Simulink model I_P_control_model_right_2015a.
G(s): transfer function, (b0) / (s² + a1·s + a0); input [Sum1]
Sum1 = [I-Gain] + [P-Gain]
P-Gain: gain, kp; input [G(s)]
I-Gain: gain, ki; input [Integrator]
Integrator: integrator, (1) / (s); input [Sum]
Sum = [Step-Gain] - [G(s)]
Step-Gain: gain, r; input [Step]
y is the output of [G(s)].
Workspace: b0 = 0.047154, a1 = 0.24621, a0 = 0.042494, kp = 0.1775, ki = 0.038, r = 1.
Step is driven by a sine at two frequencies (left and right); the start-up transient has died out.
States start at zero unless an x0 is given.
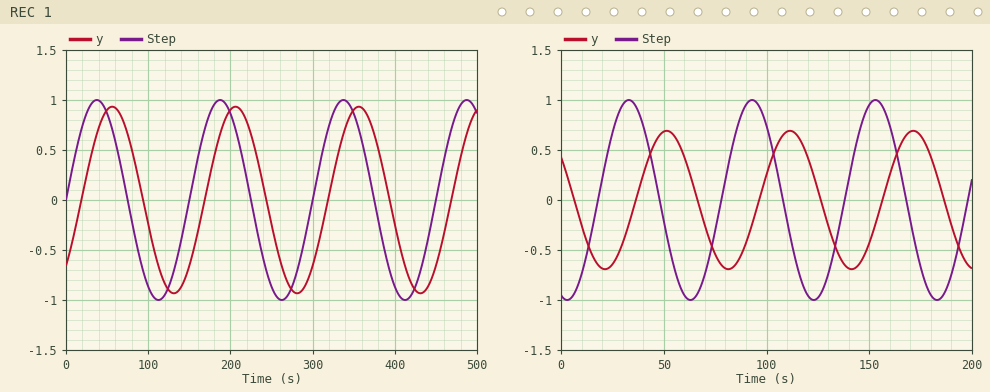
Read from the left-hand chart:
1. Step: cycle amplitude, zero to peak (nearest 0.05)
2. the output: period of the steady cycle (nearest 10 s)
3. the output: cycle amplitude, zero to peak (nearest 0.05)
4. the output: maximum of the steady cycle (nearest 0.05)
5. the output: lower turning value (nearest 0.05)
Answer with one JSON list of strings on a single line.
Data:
["1.00", "150 s", "0.95", "0.95", "-0.95"]
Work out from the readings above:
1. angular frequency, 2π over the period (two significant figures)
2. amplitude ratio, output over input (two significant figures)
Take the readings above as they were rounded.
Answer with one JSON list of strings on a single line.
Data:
["0.042 rad/s", "0.95"]
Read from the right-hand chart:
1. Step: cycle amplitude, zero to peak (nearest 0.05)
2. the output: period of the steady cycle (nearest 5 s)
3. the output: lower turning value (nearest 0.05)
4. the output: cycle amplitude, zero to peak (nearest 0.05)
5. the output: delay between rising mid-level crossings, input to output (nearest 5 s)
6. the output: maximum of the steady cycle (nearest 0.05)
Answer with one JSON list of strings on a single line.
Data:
["1.00", "60 s", "-0.70", "0.70", "20 s", "0.70"]
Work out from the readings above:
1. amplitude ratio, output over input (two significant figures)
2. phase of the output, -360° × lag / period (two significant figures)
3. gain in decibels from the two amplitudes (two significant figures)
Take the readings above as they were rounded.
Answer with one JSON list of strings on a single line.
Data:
["0.70", "-120°", "-3.1 dB"]
